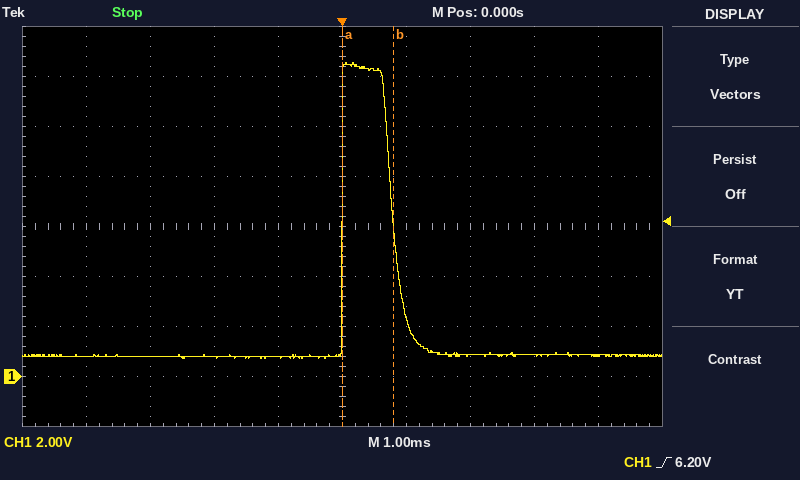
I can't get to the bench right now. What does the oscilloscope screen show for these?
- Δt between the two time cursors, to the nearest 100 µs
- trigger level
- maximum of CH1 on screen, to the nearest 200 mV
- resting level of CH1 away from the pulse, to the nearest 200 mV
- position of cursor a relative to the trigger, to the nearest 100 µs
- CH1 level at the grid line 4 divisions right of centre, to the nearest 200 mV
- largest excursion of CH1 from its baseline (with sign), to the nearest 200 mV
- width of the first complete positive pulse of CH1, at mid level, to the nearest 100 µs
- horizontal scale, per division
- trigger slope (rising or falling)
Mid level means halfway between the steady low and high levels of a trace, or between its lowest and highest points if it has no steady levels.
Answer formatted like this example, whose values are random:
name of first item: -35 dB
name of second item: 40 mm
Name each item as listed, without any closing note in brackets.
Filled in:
Δt between the two time cursors, to the nearest 100 µs: 800 µs
trigger level: 6.20 V
maximum of CH1 on screen, to the nearest 200 mV: 12.6 V
resting level of CH1 away from the pulse, to the nearest 200 mV: 800 mV
position of cursor a relative to the trigger, to the nearest 100 µs: 0.0 ms
CH1 level at the grid line 4 divisions right of centre, to the nearest 200 mV: 800 mV
largest excursion of CH1 from its baseline (with sign), to the nearest 200 mV: +11.8 V
width of the first complete positive pulse of CH1, at mid level, to the nearest 100 µs: 800 µs
horizontal scale, per division: 1 ms
trigger slope: rising
